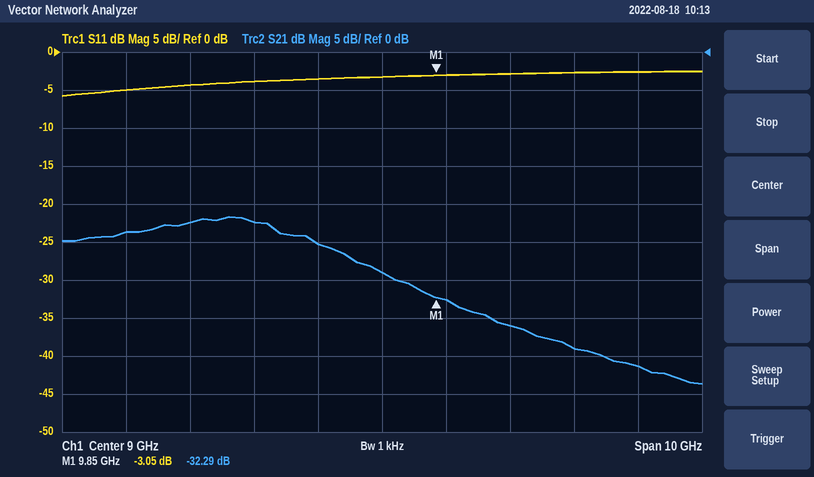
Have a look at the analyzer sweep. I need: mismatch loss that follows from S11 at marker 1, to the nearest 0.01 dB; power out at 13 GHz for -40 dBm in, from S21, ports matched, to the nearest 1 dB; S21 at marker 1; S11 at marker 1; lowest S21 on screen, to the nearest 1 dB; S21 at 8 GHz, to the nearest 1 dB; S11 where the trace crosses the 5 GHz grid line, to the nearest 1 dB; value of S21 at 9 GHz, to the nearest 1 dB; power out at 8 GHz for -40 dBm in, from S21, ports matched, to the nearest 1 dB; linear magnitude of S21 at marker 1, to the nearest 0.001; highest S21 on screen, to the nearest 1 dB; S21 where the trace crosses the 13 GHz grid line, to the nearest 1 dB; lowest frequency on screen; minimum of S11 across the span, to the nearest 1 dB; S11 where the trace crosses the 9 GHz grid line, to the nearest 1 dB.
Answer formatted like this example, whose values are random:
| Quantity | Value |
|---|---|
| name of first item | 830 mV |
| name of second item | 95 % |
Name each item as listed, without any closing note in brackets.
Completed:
| Quantity | Value |
|---|---|
| mismatch loss that follows from S11 at marker 1, to the nearest 0.01 dB | 2.97 dB |
| power out at 13 GHz for -40 dBm in, from S21, ports matched, to the nearest 1 dB | -81 dBm |
| S21 at marker 1 | -32.29 dB |
| S11 at marker 1 | -3.05 dB |
| lowest S21 on screen, to the nearest 1 dB | -44 dB |
| S21 at 8 GHz, to the nearest 1 dB | -25 dB |
| S11 where the trace crosses the 5 GHz grid line, to the nearest 1 dB | -5 dB |
| value of S21 at 9 GHz, to the nearest 1 dB | -29 dB |
| power out at 8 GHz for -40 dBm in, from S21, ports matched, to the nearest 1 dB | -65 dBm |
| linear magnitude of S21 at marker 1, to the nearest 0.001 | 0.024 |
| highest S21 on screen, to the nearest 1 dB | -22 dB |
| S21 where the trace crosses the 13 GHz grid line, to the nearest 1 dB | -41 dB |
| lowest frequency on screen | 4 GHz |
| minimum of S11 across the span, to the nearest 1 dB | -6 dB |
| S11 where the trace crosses the 9 GHz grid line, to the nearest 1 dB | -3 dB |
